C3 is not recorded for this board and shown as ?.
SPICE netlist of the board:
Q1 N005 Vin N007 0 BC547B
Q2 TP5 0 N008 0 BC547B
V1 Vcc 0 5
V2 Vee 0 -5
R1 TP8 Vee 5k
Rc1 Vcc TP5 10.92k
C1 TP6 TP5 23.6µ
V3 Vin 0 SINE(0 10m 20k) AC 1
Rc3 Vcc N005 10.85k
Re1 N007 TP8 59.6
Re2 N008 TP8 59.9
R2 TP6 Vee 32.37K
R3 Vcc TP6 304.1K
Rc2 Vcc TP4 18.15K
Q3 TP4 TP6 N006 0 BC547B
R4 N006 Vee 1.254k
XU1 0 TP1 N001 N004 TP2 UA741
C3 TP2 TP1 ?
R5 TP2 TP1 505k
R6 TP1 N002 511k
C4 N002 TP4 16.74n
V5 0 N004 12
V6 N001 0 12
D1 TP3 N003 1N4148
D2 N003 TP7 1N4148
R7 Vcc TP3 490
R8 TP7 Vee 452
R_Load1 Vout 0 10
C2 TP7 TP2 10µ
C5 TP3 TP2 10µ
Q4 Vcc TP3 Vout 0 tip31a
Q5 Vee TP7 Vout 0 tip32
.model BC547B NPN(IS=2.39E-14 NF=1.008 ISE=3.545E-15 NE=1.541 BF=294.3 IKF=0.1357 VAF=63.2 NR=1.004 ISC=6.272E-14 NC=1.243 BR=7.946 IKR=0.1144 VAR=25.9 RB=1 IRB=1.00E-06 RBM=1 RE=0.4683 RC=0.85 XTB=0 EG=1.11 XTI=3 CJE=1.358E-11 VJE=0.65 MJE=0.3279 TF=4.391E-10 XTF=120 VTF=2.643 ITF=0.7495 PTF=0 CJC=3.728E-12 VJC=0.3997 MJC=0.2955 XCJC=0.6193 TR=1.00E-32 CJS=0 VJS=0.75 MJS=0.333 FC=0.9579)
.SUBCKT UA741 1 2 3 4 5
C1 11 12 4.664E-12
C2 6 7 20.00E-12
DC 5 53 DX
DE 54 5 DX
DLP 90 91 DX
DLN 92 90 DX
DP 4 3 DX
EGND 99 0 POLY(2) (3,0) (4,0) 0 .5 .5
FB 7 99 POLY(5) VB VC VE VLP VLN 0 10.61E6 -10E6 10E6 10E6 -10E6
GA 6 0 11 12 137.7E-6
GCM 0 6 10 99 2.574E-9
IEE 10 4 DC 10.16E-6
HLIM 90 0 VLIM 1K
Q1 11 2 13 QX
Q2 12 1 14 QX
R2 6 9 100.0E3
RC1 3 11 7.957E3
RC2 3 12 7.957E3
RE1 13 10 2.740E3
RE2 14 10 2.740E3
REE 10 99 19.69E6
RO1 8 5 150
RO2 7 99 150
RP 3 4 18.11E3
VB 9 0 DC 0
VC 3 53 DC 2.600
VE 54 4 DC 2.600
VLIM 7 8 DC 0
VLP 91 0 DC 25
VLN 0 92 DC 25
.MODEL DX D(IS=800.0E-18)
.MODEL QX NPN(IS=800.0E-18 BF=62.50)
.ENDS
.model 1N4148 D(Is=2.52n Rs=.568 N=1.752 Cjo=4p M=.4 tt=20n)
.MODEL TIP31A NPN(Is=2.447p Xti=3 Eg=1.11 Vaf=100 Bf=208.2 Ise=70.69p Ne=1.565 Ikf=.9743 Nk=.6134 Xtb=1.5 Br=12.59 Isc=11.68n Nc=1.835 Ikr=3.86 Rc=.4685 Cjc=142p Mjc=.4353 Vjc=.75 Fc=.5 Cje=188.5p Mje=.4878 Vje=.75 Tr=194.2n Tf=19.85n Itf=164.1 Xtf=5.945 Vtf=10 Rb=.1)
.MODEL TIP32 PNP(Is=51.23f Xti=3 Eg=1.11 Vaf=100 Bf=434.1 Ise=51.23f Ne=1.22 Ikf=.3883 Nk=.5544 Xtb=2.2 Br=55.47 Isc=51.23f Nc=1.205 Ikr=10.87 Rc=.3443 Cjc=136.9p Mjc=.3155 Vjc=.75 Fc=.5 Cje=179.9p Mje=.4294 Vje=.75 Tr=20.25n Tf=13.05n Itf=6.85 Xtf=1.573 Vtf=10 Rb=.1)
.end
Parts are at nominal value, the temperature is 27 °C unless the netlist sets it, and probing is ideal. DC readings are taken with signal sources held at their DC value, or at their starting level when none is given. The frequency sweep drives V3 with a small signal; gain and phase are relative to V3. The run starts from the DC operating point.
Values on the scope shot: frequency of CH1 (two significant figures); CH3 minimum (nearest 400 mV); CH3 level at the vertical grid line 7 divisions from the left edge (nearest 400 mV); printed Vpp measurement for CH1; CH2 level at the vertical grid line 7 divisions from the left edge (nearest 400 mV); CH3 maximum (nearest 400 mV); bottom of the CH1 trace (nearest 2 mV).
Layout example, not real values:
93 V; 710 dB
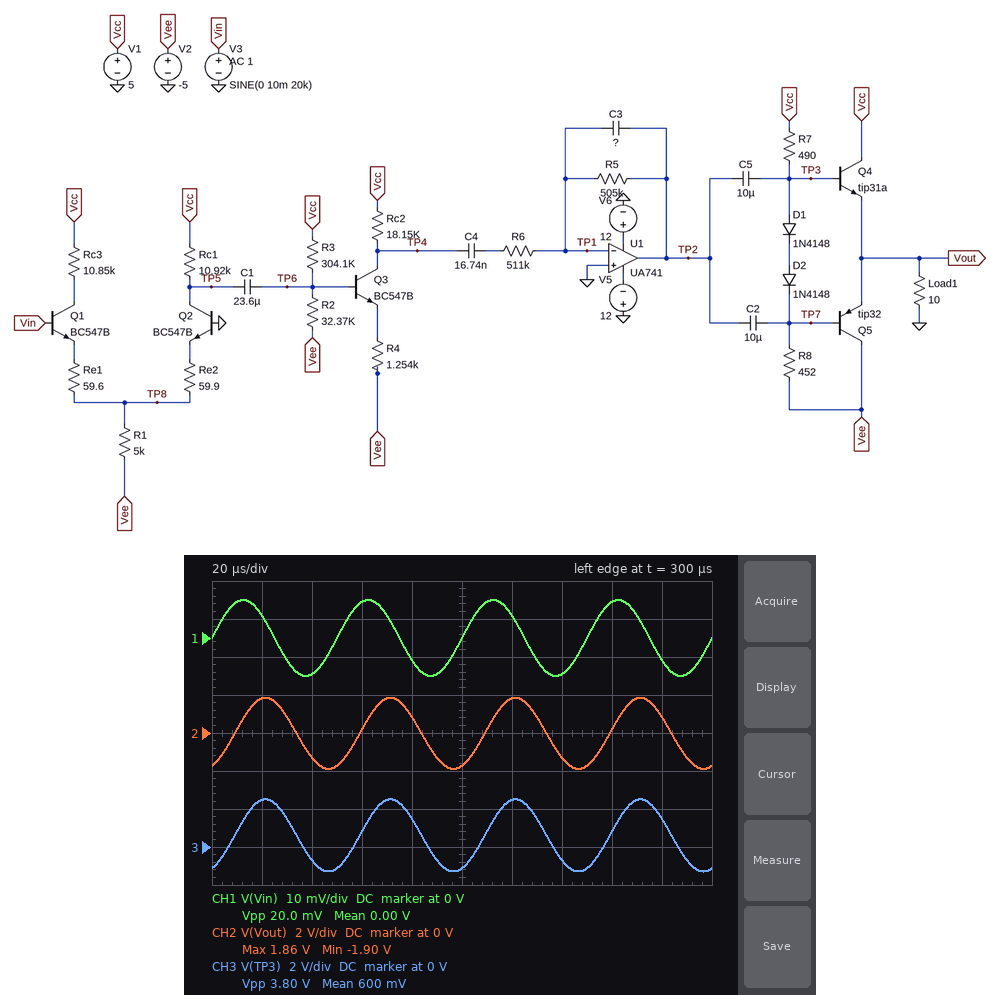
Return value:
20 kHz; -1.2 V; -800 mV; 20.0 mV; -1.2 V; 2.4 V; -10 mV
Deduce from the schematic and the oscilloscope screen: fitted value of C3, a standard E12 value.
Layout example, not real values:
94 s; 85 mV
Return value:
27 pF
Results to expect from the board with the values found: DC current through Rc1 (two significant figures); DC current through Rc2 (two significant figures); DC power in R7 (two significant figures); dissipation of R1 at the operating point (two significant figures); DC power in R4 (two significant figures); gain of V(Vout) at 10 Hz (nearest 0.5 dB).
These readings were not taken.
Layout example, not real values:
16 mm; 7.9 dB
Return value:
430 µA; 270 µA; 41 mW; 3.8 mW; 89 µW; 33.0 dB
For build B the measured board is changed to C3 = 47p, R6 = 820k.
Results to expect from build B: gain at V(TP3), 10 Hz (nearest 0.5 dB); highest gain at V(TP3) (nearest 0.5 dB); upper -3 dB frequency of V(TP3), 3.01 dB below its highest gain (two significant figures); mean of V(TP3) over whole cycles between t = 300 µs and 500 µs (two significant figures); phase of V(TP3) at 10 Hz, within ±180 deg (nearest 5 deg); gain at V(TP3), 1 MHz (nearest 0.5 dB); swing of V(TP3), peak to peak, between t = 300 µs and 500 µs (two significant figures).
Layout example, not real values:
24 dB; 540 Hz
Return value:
31.5 dB; 48.0 dB; 6.7 kHz; 570 mV; 125 deg; -6.0 dB; 1.5 V
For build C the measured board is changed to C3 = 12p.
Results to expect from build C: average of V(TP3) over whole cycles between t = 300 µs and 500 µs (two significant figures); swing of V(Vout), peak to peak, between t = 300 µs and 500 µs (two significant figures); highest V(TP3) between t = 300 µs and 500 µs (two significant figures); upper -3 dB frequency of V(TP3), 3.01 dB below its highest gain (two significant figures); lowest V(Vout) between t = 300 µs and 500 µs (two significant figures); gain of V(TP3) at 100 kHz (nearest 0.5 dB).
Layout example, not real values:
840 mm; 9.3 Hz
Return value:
580 mV; 5.7 V; 3.5 V; 25 kHz; -2.8 V; 39.5 dB
